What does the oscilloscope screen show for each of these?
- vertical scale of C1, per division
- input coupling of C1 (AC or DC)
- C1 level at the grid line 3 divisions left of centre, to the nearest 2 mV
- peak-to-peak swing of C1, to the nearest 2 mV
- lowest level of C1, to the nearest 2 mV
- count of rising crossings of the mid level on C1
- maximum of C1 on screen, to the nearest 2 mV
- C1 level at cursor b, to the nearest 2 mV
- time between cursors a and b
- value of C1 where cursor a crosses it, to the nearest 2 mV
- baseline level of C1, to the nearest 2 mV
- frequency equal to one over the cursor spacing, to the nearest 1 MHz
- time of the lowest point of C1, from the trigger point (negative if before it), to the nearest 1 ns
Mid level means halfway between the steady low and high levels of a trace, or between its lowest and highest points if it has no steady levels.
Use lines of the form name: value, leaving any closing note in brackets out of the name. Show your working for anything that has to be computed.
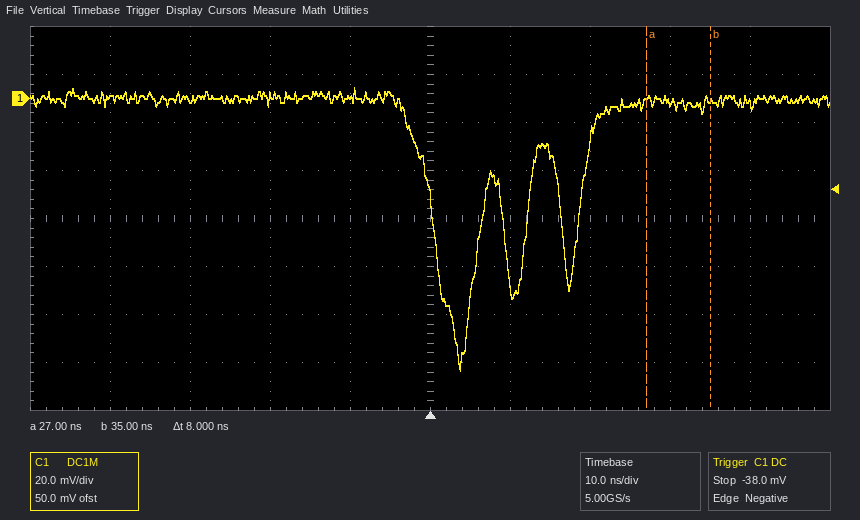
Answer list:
vertical scale of C1, per division: 20 mV
input coupling of C1: DC
C1 level at the grid line 3 divisions left of centre, to the nearest 2 mV: 0 mV
peak-to-peak swing of C1, to the nearest 2 mV: 4 mV − (-114 mV) = 118 mV
lowest level of C1, to the nearest 2 mV: -114 mV
count of rising crossings of the mid level on C1: 3
maximum of C1 on screen, to the nearest 2 mV: 4 mV
C1 level at cursor b, to the nearest 2 mV: 0 mV
time between cursors a and b: 8 ns
value of C1 where cursor a crosses it, to the nearest 2 mV: 0 mV
baseline level of C1, to the nearest 2 mV: 0 mV
frequency equal to one over the cursor spacing, to the nearest 1 MHz: 1 / 8 ns ≈ 125 MHz
time of the lowest point of C1, from the trigger point (negative if before it), to the nearest 1 ns: +4 ns
